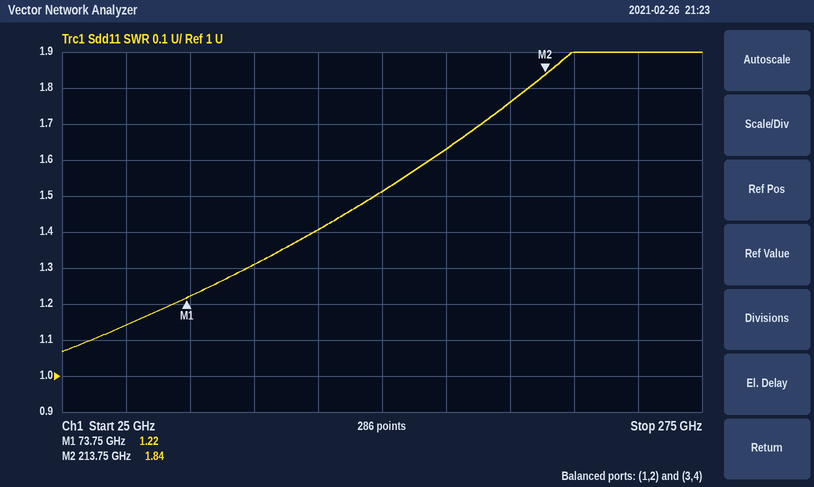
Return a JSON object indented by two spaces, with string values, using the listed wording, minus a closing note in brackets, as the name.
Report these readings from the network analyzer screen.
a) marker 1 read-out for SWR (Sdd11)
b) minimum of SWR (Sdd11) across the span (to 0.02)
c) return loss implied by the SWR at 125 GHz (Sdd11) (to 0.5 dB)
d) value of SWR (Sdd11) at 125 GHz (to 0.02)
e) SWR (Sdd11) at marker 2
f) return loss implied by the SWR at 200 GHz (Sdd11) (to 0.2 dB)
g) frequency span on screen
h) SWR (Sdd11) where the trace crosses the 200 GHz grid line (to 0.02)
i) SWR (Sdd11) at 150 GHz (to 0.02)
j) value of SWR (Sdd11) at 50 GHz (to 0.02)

{
  "marker 1 read-out for SWR": "1.22",
  "minimum of SWR (Sdd11) across the span": "1.06",
  "return loss implied by the SWR at 125 GHz (Sdd11)": "15.5 dB",
  "value of SWR (Sdd11) at 125 GHz": "1.40",
  "SWR (Sdd11) at marker 2": "1.84",
  "return loss implied by the SWR at 200 GHz (Sdd11)": "11.2 dB",
  "frequency span on screen": "250 GHz",
  "SWR (Sdd11) where the trace crosses the 200 GHz grid line": "1.76",
  "SWR (Sdd11) at 150 GHz": "1.52",
  "value of SWR (Sdd11) at 50 GHz": "1.14"
}
